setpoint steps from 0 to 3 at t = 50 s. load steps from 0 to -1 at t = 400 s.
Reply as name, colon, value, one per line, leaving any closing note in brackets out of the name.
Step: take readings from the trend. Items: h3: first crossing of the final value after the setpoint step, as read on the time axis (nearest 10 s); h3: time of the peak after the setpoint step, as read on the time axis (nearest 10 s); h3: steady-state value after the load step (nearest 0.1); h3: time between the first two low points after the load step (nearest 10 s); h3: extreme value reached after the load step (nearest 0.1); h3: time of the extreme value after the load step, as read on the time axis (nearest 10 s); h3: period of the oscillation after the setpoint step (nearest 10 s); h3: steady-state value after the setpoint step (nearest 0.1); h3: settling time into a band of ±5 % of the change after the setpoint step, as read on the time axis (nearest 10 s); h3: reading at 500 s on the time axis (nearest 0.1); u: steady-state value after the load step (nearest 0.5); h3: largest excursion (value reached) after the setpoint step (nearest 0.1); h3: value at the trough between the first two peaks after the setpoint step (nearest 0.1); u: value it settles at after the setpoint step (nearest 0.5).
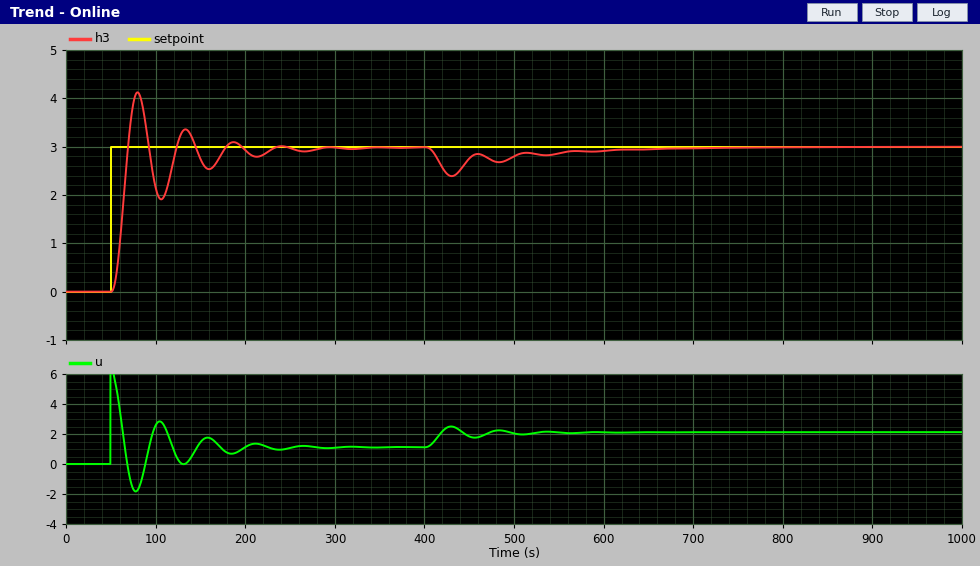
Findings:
h3: first crossing of the final value after the setpoint step, as read on the time axis: 70 s
h3: time of the peak after the setpoint step, as read on the time axis: 80 s
h3: steady-state value after the load step: 3.0
h3: time between the first two low points after the load step: 50 s
h3: extreme value reached after the load step: 2.4
h3: time of the extreme value after the load step, as read on the time axis: 430 s
h3: period of the oscillation after the setpoint step: 50 s
h3: steady-state value after the setpoint step: 3.0
h3: settling time into a band of ±5 % of the change after the setpoint step, as read on the time axis: 220 s
h3: reading at 500 s on the time axis: 2.8
u: steady-state value after the load step: 2.0
h3: largest excursion (value reached) after the setpoint step: 4.1
h3: value at the trough between the first two peaks after the setpoint step: 1.9
u: value it settles at after the setpoint step: 1.0
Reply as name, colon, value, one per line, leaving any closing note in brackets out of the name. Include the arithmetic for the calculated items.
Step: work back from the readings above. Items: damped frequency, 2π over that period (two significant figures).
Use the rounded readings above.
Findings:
damped frequency, 2π over that period: 2π / 50 = 0.13 rad/s
